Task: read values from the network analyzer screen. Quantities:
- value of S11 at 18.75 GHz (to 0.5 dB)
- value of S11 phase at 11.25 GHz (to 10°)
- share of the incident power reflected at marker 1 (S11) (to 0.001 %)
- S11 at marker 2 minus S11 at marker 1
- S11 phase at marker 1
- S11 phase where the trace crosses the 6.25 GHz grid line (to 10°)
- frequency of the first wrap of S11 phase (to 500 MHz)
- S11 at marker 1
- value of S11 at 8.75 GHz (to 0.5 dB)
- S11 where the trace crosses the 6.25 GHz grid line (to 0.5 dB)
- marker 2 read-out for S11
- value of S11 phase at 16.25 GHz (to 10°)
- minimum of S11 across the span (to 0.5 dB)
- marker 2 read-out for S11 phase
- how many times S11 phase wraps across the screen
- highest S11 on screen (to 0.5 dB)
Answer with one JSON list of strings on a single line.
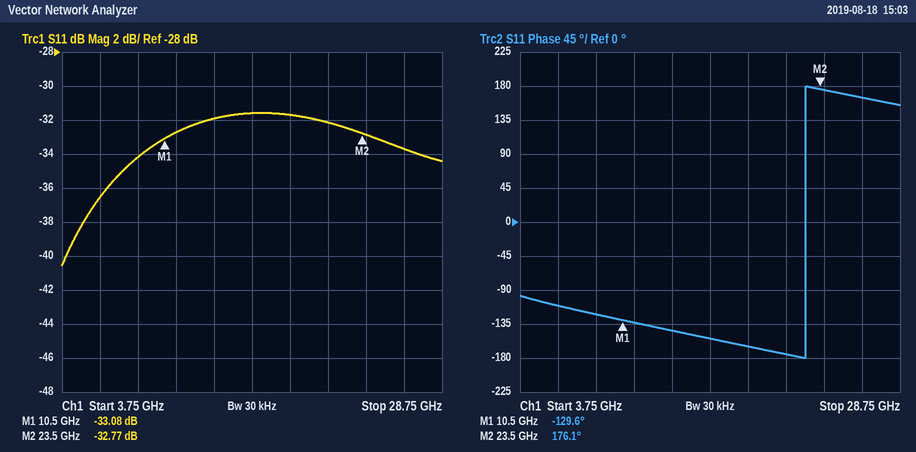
["-31.5 dB", "-130°", "0.049 %", "0.31 dB", "-129.6°", "-110°", "22.5 GHz", "-33.08 dB", "-34.0 dB", "-36.5 dB", "-32.77 dB", "-150°", "-40.5 dB", "176.1°", "1", "-31.5 dB"]
